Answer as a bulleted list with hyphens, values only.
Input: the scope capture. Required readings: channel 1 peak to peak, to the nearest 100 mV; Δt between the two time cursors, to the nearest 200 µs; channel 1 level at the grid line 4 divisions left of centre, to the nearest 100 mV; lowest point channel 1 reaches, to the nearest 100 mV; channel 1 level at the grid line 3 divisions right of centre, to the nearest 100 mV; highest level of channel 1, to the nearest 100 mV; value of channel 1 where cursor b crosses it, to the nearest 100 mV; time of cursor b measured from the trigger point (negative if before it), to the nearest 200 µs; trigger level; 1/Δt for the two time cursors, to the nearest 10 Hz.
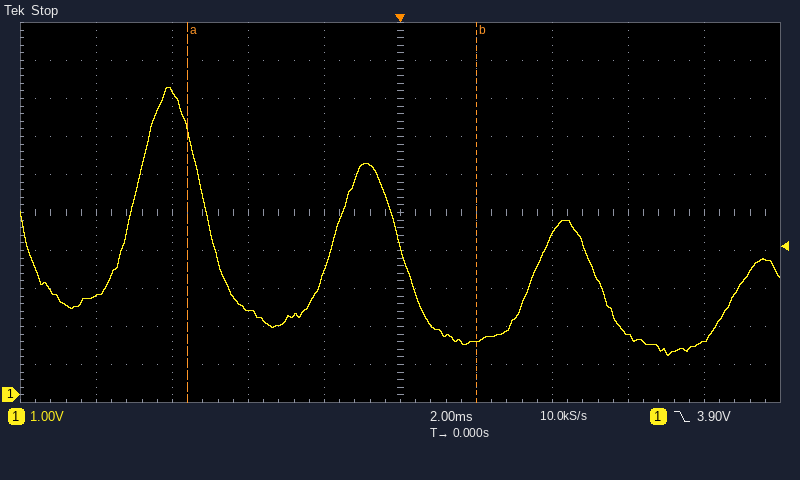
- 7.1 V
- 7.6 ms
- 2.6 V
- 1.0 V
- 1.6 V
- 8.1 V
- 1.4 V
- +2.0 ms
- 3.90 V
- 130 Hz
